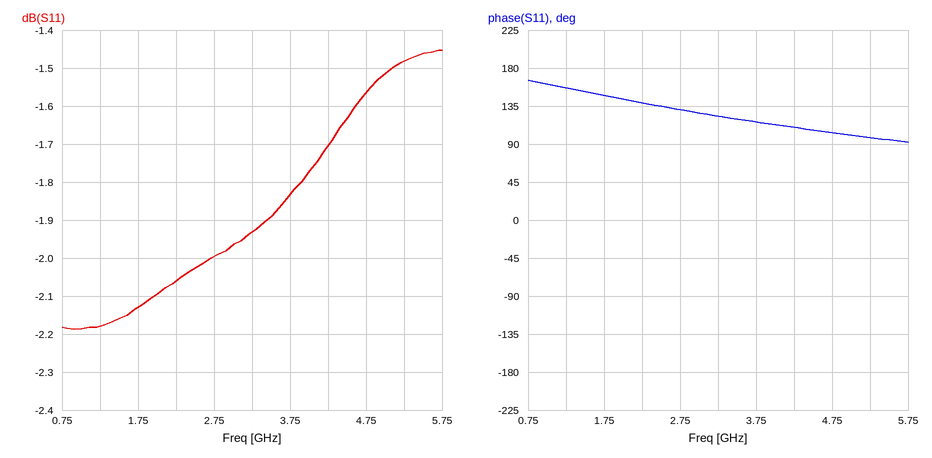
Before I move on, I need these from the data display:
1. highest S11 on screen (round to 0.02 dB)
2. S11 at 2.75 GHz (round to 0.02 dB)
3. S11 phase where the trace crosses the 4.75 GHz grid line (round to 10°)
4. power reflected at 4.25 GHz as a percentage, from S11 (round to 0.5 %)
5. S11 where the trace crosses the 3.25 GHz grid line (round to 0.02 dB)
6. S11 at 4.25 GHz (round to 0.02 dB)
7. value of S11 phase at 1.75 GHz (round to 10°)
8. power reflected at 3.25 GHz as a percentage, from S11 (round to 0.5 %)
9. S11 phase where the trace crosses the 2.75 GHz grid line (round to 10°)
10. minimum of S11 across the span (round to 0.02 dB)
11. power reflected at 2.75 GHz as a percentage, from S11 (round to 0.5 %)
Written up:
-1.46 dB
-2.00 dB
100°
67.5 %
-1.94 dB
-1.70 dB
150°
64.0 %
130°
-2.18 dB
63.0 %
